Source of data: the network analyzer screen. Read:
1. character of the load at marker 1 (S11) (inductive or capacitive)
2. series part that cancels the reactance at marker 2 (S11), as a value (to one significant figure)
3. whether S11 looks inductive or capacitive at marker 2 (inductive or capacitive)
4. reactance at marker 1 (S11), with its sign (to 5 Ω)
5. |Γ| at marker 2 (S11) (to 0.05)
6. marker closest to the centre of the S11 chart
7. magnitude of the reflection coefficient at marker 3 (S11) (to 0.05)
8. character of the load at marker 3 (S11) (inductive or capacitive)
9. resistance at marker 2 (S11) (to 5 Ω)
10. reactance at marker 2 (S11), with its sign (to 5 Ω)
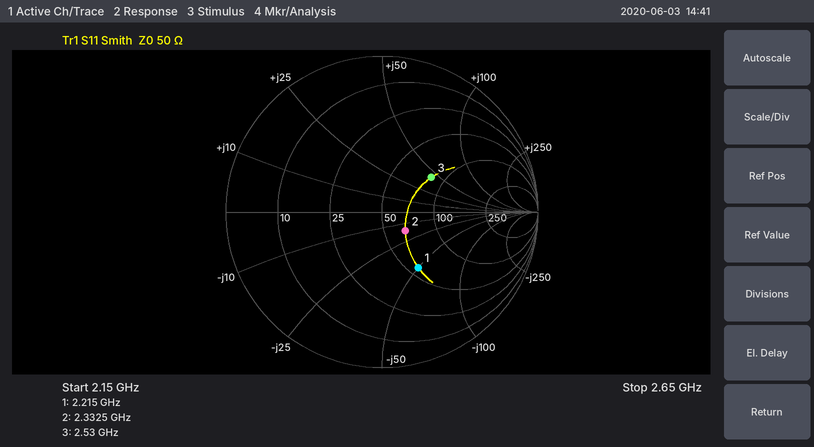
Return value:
capacitive
1 nH
capacitive
-50 Ω
0.20
marker 2
0.40
inductive
65 Ω
-15 Ω
